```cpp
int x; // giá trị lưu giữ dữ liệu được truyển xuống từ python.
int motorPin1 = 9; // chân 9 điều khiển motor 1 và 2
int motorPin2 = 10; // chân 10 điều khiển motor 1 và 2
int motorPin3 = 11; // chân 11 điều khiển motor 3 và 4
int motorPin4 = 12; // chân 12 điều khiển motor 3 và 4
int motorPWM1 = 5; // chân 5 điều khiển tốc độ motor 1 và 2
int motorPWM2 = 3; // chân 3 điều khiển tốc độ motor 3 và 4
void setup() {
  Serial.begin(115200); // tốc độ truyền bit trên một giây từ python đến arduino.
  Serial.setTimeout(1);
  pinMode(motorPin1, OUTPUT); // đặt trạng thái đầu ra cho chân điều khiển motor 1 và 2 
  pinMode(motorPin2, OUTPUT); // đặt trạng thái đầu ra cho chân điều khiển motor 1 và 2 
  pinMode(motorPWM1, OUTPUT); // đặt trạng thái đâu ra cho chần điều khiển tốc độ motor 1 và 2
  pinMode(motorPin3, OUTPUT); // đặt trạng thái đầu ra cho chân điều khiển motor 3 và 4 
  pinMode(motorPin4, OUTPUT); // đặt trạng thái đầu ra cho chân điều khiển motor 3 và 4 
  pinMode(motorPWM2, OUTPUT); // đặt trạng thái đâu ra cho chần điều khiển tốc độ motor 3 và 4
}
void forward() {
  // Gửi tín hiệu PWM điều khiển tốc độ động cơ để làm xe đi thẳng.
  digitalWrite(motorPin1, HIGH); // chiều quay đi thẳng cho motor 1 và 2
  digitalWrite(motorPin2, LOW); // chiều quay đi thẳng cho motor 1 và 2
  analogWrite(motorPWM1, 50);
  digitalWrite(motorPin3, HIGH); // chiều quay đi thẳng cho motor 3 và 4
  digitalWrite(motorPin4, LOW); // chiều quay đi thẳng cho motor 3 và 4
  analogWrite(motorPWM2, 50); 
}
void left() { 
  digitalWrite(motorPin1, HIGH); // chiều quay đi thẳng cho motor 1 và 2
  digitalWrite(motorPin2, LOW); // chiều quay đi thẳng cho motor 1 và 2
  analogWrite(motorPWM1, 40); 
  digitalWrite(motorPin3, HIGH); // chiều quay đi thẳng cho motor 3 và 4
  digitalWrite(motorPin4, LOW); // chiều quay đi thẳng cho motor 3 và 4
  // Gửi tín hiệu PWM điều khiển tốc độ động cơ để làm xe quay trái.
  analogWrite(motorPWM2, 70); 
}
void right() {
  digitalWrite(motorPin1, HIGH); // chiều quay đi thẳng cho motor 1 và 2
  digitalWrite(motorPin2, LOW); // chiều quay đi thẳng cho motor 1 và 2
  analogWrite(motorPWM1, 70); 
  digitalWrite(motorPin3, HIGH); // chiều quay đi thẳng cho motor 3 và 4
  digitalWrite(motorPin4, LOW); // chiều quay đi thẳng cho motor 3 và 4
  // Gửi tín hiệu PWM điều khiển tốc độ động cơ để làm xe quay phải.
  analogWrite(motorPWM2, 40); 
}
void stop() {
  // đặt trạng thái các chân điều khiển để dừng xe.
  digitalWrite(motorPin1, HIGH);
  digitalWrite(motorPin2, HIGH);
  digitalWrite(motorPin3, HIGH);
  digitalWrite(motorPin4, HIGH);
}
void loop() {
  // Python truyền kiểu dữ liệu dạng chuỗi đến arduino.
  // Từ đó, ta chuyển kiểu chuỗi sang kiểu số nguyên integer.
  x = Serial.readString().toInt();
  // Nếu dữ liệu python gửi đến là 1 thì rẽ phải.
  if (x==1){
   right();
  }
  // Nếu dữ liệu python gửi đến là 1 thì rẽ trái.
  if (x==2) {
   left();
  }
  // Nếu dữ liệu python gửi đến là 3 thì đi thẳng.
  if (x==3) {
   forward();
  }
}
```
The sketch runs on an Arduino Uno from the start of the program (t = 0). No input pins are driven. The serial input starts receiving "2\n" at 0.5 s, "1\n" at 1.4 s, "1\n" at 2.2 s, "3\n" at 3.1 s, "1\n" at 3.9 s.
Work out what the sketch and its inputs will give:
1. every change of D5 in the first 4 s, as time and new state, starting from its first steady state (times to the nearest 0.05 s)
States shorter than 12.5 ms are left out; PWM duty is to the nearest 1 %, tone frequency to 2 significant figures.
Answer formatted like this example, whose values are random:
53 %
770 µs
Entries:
0 s low; 0.5 s PWM 16 %; 1.4 s PWM 28 %; 3.1 s PWM 20 %; 3.9 s PWM 28 %
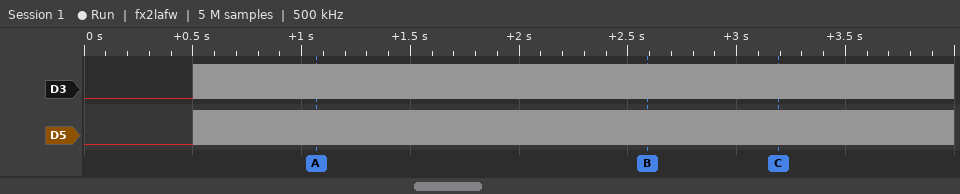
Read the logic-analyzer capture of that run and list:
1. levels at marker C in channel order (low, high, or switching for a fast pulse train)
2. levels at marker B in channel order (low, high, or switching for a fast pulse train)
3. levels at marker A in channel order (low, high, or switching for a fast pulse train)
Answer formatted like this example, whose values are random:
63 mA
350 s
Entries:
D3 switching, D5 switching
D3 switching, D5 switching
D3 switching, D5 switching
